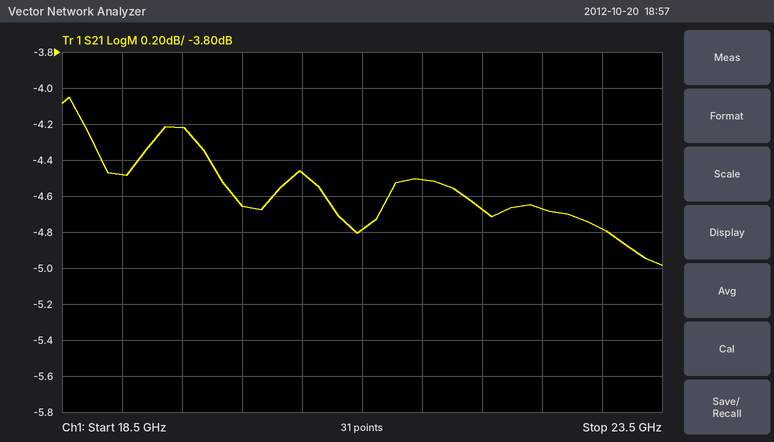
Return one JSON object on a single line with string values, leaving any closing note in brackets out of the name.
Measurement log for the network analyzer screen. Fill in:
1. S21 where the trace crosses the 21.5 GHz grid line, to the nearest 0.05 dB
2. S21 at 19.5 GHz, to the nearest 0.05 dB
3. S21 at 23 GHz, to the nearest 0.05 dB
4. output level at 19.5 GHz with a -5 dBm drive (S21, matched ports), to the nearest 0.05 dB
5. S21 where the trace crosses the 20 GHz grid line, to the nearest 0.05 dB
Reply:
{"S21 where the trace crosses the 21.5 GHz grid line, to the nearest 0.05 dB": "-4.50 dB", "S21 at 19.5 GHz, to the nearest 0.05 dB": "-4.20 dB", "S21 at 23 GHz, to the nearest 0.05 dB": "-4.80 dB", "output level at 19.5 GHz with a -5 dBm drive (S21, matched ports), to the nearest 0.05 dB": "-9.20 dBm", "S21 where the trace crosses the 20 GHz grid line, to the nearest 0.05 dB": "-4.65 dB"}
